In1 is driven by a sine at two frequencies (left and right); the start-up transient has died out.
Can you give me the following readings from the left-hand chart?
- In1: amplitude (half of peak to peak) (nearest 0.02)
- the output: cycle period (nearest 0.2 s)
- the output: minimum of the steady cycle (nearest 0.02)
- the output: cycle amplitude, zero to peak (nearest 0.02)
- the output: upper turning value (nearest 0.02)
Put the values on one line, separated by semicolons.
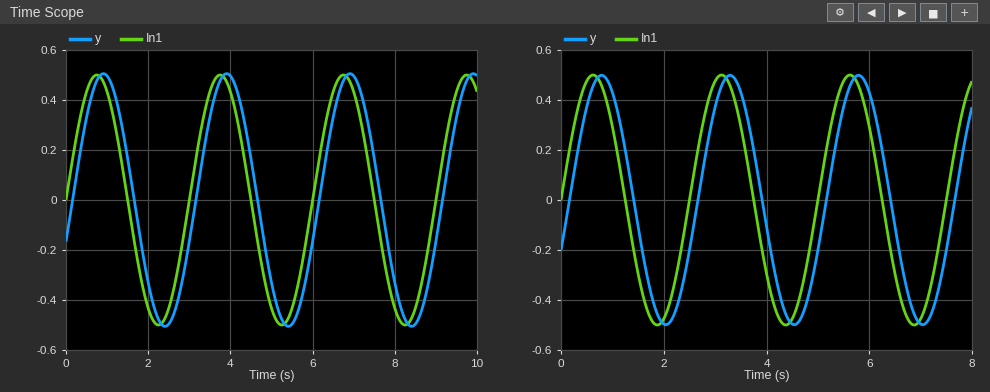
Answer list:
0.50; 3.0 s; -0.50; 0.50; 0.50
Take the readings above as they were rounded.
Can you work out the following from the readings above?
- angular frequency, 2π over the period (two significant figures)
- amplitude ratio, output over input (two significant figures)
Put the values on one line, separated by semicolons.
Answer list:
2.1 rad/s; 1.0
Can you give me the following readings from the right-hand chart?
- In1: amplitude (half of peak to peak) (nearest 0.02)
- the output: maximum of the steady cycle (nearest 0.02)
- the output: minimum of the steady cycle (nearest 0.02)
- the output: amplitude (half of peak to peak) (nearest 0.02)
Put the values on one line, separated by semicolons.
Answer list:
0.50; 0.50; -0.50; 0.50
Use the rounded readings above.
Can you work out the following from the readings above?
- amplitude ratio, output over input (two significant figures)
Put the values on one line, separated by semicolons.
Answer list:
1.0
